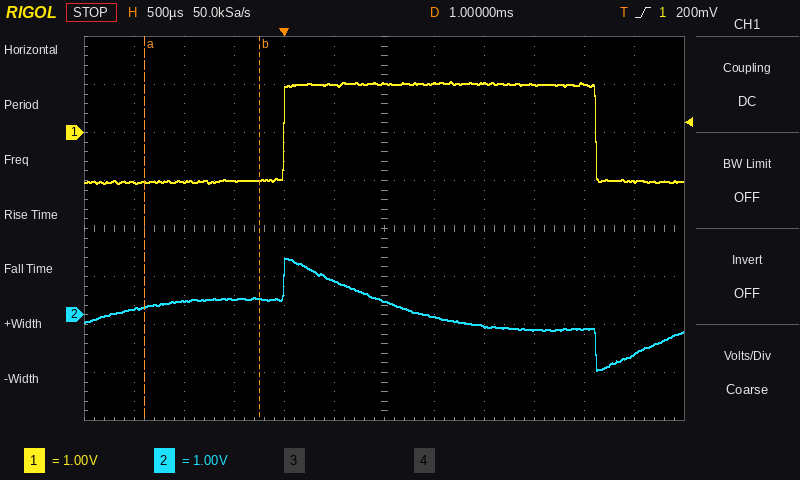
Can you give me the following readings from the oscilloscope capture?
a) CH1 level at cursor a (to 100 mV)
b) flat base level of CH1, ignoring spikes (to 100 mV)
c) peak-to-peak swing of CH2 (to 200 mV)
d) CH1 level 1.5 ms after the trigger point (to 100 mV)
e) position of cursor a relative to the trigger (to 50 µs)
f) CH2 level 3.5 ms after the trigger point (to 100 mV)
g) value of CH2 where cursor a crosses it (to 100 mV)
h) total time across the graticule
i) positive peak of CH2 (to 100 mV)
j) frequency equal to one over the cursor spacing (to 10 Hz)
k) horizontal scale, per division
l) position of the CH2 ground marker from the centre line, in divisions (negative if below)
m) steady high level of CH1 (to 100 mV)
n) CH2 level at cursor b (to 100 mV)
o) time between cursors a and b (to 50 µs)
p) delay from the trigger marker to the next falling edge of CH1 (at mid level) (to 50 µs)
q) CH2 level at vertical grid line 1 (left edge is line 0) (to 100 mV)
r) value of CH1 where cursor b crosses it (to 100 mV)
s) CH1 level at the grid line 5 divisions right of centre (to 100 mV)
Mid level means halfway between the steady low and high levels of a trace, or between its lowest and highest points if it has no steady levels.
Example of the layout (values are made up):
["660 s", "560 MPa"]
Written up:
["-1.0 V", "-1.0 V", "2.4 V", "1.0 V", "-1.40 ms", "-800 mV", "200 mV", "6 ms", "1.2 V", "870 Hz", "500 µs", "-1.8 div", "1.0 V", "300 mV", "1.15 ms", "3.10 ms", "100 mV", "-1.0 V", "-1.0 V"]
